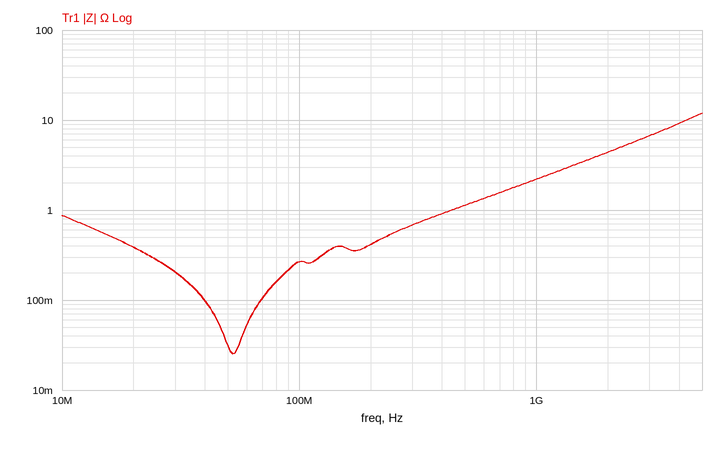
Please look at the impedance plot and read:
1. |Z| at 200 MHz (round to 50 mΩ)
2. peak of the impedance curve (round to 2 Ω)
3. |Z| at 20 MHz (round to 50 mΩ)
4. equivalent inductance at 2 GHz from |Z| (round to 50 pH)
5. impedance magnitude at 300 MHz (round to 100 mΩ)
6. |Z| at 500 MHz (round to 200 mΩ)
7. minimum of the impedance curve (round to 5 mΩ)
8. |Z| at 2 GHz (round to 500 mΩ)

400 mΩ
12 Ω
400 mΩ
350 pH
700 mΩ
1.2 Ω
25 mΩ
4.5 Ω
